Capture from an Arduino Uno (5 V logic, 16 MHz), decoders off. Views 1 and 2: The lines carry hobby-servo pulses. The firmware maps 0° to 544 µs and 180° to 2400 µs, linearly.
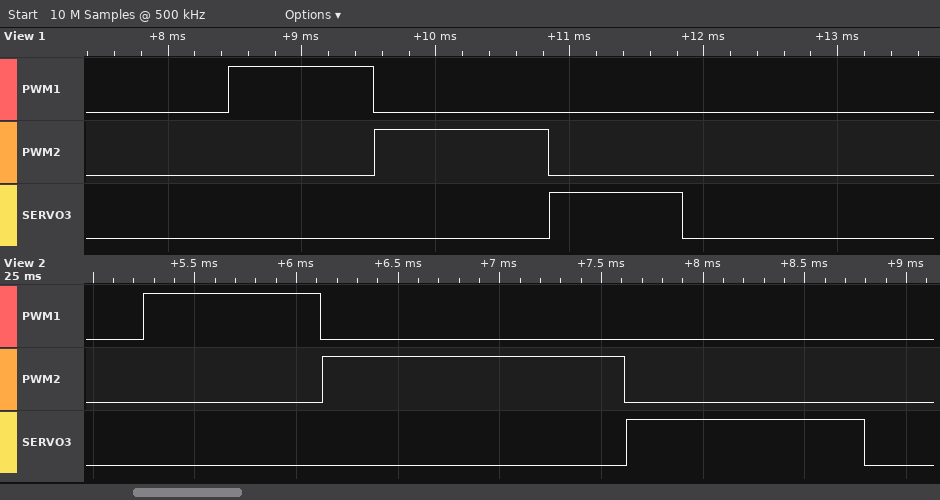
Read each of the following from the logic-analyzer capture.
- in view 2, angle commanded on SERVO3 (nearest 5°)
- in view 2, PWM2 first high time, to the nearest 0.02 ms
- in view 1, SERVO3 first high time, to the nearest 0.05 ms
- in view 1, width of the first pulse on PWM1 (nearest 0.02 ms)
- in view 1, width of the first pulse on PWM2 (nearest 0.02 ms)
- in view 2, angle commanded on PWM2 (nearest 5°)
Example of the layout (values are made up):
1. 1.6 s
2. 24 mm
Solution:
1. 60°
2. 1.48 ms
3. 1.00 ms
4. 1.08 ms
5. 1.30 ms
6. 90°
